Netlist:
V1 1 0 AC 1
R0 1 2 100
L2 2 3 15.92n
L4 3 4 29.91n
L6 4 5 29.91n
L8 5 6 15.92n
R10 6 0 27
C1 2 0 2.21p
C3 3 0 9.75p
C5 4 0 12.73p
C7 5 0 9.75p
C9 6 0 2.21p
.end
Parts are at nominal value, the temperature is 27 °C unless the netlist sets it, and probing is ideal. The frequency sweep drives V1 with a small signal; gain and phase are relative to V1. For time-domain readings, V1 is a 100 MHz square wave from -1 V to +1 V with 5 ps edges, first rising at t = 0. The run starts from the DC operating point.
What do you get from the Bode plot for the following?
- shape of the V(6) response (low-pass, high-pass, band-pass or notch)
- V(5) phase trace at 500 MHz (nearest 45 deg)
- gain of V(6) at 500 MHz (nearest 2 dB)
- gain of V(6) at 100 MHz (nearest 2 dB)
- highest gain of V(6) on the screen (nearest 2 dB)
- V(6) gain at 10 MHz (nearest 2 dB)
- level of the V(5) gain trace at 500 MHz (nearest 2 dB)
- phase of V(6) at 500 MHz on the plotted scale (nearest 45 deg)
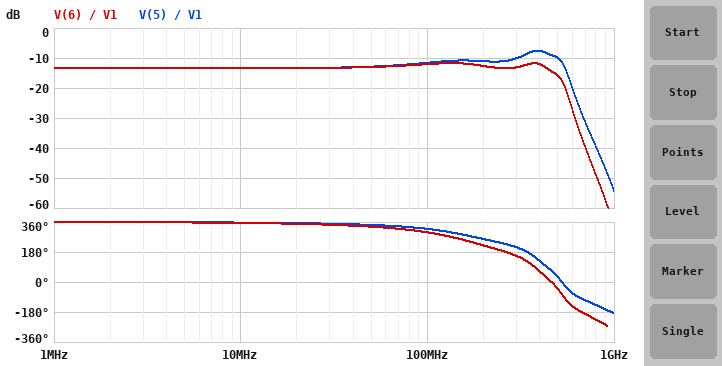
low-pass
45 deg
-16 dB
-12 dB
-12 dB
-14 dB
-10 dB
-45 deg
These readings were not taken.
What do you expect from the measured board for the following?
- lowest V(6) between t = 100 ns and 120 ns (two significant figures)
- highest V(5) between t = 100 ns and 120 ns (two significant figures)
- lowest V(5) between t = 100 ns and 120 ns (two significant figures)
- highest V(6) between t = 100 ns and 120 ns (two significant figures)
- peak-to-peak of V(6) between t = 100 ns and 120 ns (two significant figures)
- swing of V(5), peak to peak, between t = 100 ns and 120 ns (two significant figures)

-340 mV
450 mV
-450 mV
340 mV
680 mV
890 mV
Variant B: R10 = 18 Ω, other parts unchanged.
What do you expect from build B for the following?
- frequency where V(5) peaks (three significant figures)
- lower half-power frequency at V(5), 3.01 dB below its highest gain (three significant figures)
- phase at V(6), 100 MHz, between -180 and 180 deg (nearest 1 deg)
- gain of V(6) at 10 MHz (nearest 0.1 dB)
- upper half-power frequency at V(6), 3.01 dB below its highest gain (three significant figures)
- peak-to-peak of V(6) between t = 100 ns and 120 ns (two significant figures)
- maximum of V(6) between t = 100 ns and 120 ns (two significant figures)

384 MHz
314 MHz
-59 deg
-16.3 dB
444 MHz
530 mV
270 mV
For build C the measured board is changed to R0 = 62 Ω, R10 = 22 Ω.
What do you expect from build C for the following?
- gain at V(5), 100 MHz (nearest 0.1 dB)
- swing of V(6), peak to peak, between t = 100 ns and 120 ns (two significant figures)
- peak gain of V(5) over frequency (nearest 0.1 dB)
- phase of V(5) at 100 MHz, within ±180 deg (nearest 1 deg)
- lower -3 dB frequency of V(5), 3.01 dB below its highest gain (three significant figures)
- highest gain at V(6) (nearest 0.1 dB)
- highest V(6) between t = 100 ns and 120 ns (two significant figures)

-10.3 dB
760 mV
-5.5 dB
-40 deg
240 MHz
-10.9 dB
380 mV
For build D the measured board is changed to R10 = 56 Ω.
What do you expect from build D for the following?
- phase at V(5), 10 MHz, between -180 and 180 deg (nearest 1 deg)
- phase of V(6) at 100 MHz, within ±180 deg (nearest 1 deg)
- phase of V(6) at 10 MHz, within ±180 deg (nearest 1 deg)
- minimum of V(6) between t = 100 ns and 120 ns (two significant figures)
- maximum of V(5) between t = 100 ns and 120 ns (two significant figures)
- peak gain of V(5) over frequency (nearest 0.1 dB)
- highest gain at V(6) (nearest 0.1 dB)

-6 deg
-67 deg
-7 deg
-470 mV
470 mV
-8.2 dB
-8.7 dB
